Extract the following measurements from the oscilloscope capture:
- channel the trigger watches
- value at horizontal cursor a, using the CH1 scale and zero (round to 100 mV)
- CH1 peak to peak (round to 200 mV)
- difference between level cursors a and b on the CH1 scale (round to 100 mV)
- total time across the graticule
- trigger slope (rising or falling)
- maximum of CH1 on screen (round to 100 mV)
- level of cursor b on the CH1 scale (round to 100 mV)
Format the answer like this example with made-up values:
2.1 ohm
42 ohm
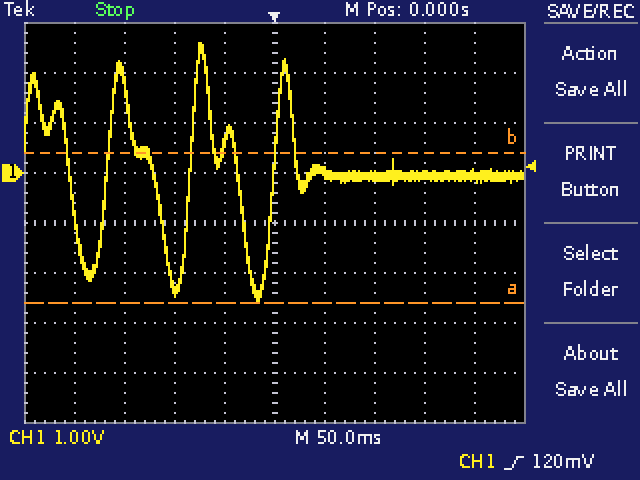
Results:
CH1
-2.6 V
5.2 V
3.0 V
500 ms
rising
2.6 V
400 mV
